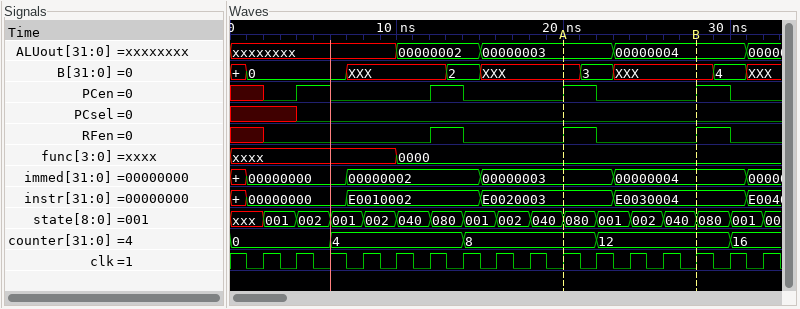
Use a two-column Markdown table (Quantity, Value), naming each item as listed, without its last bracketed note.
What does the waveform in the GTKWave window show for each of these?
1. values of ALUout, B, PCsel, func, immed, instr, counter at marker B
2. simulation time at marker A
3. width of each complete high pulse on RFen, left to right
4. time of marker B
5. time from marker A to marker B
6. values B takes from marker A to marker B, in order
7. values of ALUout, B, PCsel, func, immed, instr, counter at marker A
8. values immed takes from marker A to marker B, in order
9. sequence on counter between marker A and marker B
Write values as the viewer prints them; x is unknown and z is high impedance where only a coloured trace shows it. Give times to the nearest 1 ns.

| Quantity | Value |
|---|---|
| values of ALUout, B, PCsel, func, immed, instr, counter at marker B | ALUout=00000004, B=XXX, PCsel=0, func=0000, immed=00000004, instr=E0030004, counter=12 |
| simulation time at marker A | 20 ns |
| width of each complete high pulse on RFen, left to right | 2 ns, 2 ns, 2 ns |
| time of marker B | 28 ns |
| time from marker A to marker B | 8 ns |
| values B takes from marker A to marker B, in order | XXX, 3, XXX |
| values of ALUout, B, PCsel, func, immed, instr, counter at marker A | ALUout=00000003, B=XXX, PCsel=0, func=0000, immed=00000003, instr=E0020003, counter=8 |
| values immed takes from marker A to marker B, in order | 00000003, 00000004 |
| sequence on counter between marker A and marker B | 8, 12 |
